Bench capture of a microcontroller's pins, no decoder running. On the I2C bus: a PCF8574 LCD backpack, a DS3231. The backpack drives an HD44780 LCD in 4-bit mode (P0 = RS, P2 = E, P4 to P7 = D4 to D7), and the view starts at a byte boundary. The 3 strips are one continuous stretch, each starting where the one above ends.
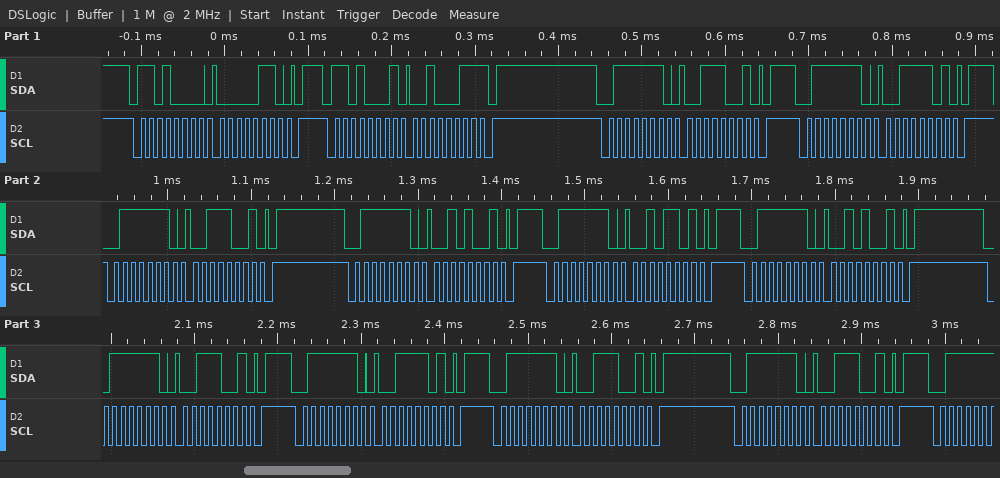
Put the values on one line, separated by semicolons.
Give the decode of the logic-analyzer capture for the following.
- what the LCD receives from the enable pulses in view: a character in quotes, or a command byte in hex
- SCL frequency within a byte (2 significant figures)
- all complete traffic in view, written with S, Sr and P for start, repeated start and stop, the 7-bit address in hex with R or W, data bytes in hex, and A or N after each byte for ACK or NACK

'2'; 100 kHz; S 68W A 06 A P S 68R A 23 N P S 3FW A 39 A P S 3FW A 3D A P S 3FW A 39 A P S 3FW A 29 A P S 3FW A 2D A P S 3FW A 29 A P S 3FW A 39 A P S 3FW A 3D A P S 3FW A 39 A P S 3FW A 39 A P
